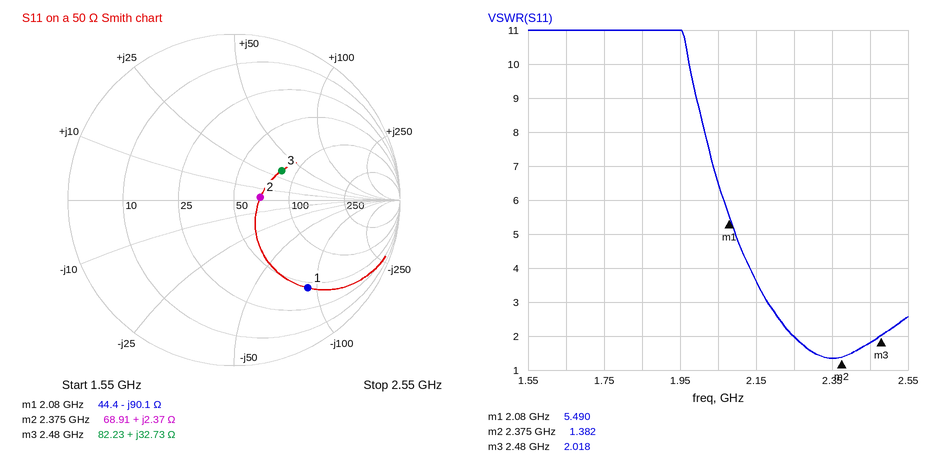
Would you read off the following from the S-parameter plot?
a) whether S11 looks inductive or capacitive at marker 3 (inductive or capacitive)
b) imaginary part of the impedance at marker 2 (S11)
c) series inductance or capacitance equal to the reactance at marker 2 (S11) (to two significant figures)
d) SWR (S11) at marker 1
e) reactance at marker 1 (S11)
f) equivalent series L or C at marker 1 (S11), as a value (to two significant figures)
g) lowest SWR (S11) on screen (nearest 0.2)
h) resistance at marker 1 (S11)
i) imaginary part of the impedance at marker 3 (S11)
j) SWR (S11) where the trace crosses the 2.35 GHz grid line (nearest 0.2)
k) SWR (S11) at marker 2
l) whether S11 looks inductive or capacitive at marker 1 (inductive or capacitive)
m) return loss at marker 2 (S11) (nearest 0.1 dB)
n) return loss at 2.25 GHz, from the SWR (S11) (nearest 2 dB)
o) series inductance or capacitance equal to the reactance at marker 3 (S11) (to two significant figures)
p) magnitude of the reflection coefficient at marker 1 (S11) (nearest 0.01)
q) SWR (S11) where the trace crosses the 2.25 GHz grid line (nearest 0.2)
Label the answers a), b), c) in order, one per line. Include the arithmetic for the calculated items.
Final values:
a) inductive
b) +2.37 Ω
c) L = 2.37 Ω/(2π × 2.375 GHz) ≈ 159 pH, so 160 pH to two significant figures
d) 5.490
e) -90.1 Ω
f) C = 1/(2π × 2.08 GHz × 90.1 Ω) ≈ 849 fF, so 850 fF to two significant figures
g) 1.4
h) 44.4 Ω
i) +32.73 Ω
j) 1.4
k) 1.382
l) capacitive
m) 15.9 dB
n) −20 log10((2 − 1)/(2 + 1)) ≈ 10 dB
o) L = 32.73 Ω/(2π × 2.48 GHz) ≈ 2.1 nH
p) 0.69
q) 2.0
